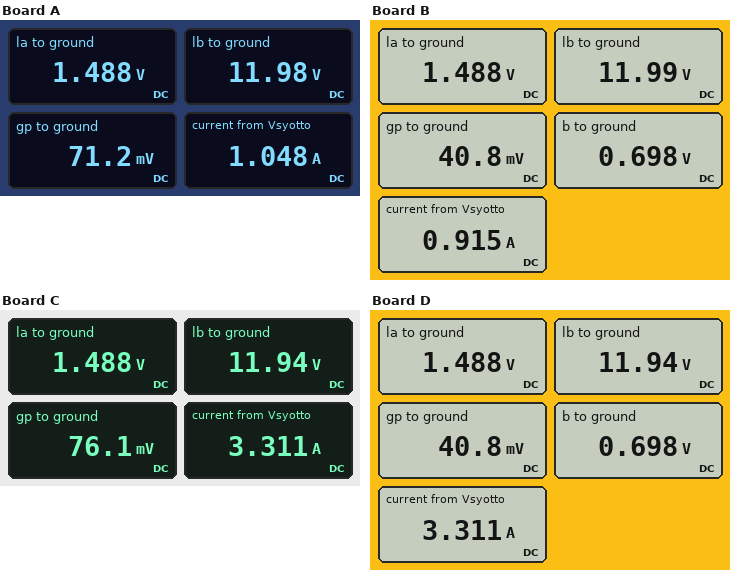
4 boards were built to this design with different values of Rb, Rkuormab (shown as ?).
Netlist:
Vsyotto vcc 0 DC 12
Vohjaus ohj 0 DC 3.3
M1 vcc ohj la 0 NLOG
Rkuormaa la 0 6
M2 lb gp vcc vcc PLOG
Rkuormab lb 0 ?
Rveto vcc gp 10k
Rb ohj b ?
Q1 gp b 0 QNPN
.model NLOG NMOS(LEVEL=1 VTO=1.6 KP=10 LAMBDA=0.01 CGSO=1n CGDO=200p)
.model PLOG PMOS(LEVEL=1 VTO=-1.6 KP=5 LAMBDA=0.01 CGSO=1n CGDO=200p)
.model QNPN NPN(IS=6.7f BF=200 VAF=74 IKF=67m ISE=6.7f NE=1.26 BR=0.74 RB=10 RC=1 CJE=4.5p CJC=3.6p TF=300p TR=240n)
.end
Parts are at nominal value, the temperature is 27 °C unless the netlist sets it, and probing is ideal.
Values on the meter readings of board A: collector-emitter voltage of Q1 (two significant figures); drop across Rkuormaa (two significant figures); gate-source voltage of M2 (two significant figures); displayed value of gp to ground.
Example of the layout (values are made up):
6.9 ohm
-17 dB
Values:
71 mV
1.5 V
-12 V
71.2 mV
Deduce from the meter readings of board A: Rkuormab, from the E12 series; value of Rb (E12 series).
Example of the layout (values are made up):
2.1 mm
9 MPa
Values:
15 Ω
18 kΩ
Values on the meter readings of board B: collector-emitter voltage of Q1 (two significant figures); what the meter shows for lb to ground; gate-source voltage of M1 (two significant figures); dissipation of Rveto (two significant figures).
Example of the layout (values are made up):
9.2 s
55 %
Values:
41 mV
11.99 V
1.8 V
14 mW
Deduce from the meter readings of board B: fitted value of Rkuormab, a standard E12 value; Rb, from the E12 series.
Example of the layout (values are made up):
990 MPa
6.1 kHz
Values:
18 Ω
3.3 kΩ
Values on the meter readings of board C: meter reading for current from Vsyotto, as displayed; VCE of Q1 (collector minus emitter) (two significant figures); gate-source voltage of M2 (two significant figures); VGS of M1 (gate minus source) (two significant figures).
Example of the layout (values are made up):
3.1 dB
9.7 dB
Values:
3.311 A
76 mV
-12 V
1.8 V
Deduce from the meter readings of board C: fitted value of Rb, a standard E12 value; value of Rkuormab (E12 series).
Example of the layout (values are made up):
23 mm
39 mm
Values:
22 kΩ
3.9 Ω
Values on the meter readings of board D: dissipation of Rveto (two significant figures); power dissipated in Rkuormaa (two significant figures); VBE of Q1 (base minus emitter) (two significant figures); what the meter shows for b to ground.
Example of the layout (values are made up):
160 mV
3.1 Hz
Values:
14 mW
370 mW
700 mV
0.698 V
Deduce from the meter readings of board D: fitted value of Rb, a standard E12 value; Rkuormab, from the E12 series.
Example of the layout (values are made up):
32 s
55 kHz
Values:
3.3 kΩ
3.9 Ω
